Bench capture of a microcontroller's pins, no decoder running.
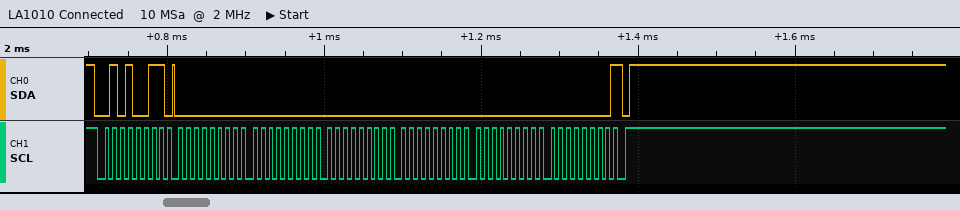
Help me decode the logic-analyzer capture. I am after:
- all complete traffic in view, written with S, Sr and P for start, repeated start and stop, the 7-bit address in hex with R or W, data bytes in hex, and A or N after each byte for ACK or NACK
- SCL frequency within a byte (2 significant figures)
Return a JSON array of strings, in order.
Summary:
["S 29R A 00 A 00 A 00 A 00 A 00 A 00 N P", "100 kHz"]
